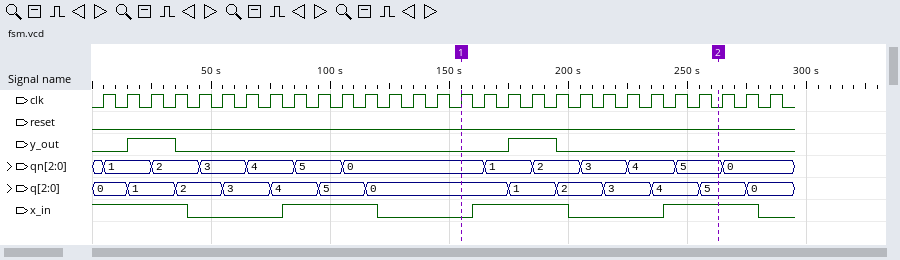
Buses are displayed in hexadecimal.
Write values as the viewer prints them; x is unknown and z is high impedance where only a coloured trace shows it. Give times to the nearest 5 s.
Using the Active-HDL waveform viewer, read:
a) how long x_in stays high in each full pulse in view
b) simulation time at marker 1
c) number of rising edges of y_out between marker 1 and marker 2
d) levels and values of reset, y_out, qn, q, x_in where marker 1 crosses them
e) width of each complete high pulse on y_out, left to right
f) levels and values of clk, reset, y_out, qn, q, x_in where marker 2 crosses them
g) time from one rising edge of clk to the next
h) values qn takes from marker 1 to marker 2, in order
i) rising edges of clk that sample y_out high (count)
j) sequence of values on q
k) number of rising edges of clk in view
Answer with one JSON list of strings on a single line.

["40 s, 40 s, 40 s", "155 s", "1", "reset=0, y_out=0, qn=0, q=0, x_in=0", "20 s, 20 s", "clk=0, reset=0, y_out=0, qn=5, q=5, x_in=1", "10 s", "0, 1, 2, 3, 4, 5", "4", "0, 1, 2, 3, 4, 5, 0, 1, 2, 3, 4, 5, 0", "29"]
